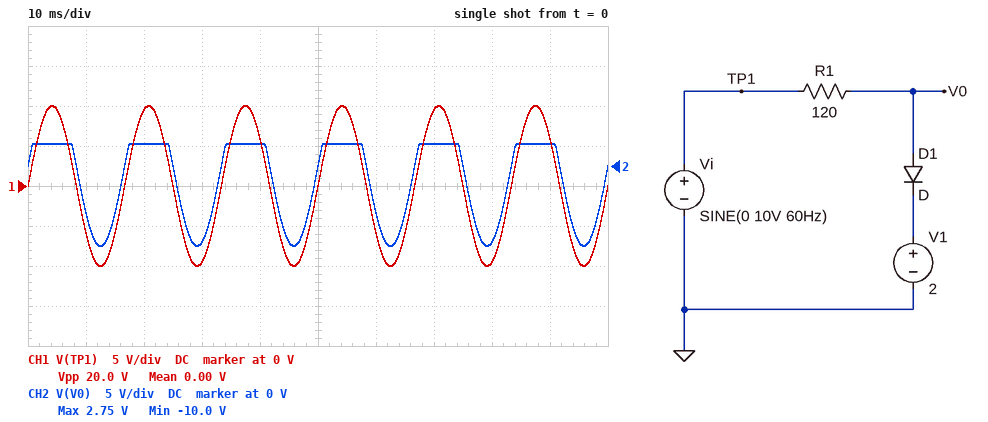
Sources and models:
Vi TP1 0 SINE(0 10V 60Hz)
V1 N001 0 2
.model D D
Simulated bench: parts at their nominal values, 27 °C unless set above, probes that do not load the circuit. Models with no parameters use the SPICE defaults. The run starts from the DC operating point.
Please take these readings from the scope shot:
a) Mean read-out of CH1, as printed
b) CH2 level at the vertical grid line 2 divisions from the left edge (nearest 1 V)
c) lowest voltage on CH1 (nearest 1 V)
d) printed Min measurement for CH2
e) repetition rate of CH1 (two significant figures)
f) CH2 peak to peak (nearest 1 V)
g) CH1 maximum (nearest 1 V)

0.00 V
3 V
-10 V
-10.0 V
60 Hz
13 V
10 V
